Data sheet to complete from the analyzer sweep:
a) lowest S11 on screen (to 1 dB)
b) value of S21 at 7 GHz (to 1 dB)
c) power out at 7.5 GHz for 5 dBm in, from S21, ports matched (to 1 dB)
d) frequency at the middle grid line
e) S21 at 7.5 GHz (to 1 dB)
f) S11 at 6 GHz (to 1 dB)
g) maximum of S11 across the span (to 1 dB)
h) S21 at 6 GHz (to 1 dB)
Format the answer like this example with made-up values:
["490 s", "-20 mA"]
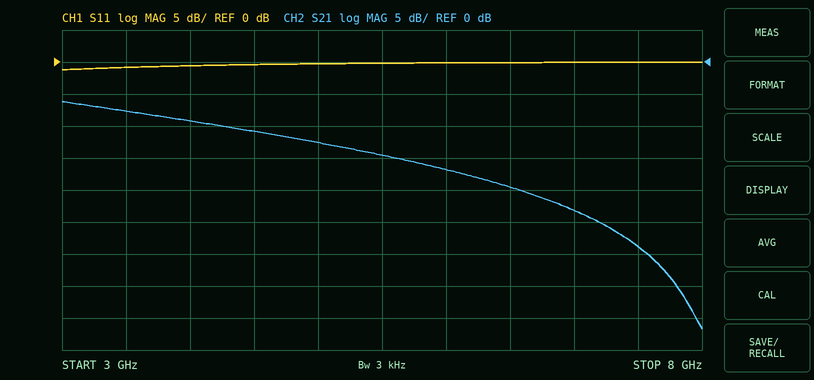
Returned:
["-1 dB", "-23 dB", "-24 dBm", "5.5 GHz", "-29 dB", "0 dB", "0 dB", "-17 dB"]
